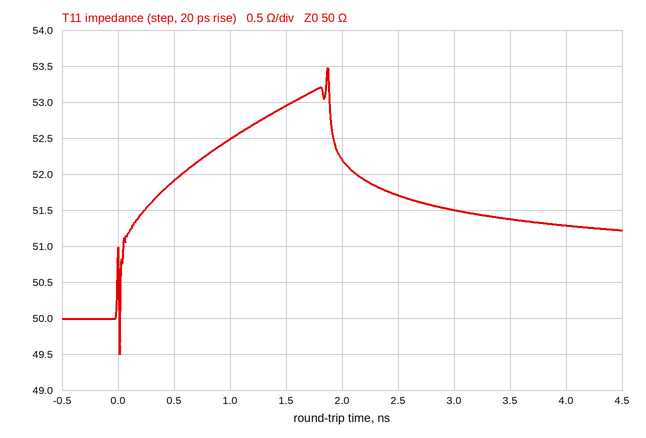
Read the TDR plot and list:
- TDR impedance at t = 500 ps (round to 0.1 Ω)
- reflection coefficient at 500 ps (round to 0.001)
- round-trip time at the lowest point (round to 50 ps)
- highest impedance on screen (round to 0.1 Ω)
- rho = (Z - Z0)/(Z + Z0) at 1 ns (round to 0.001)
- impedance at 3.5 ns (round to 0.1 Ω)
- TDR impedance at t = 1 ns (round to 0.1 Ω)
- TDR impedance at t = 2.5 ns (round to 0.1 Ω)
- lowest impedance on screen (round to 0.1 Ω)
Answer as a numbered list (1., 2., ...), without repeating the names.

1. 51.9 Ω
2. +0.019
3. 0 ps
4. 53.5 Ω
5. +0.024
6. 51.4 Ω
7. 52.5 Ω
8. 51.7 Ω
9. 49.5 Ω
